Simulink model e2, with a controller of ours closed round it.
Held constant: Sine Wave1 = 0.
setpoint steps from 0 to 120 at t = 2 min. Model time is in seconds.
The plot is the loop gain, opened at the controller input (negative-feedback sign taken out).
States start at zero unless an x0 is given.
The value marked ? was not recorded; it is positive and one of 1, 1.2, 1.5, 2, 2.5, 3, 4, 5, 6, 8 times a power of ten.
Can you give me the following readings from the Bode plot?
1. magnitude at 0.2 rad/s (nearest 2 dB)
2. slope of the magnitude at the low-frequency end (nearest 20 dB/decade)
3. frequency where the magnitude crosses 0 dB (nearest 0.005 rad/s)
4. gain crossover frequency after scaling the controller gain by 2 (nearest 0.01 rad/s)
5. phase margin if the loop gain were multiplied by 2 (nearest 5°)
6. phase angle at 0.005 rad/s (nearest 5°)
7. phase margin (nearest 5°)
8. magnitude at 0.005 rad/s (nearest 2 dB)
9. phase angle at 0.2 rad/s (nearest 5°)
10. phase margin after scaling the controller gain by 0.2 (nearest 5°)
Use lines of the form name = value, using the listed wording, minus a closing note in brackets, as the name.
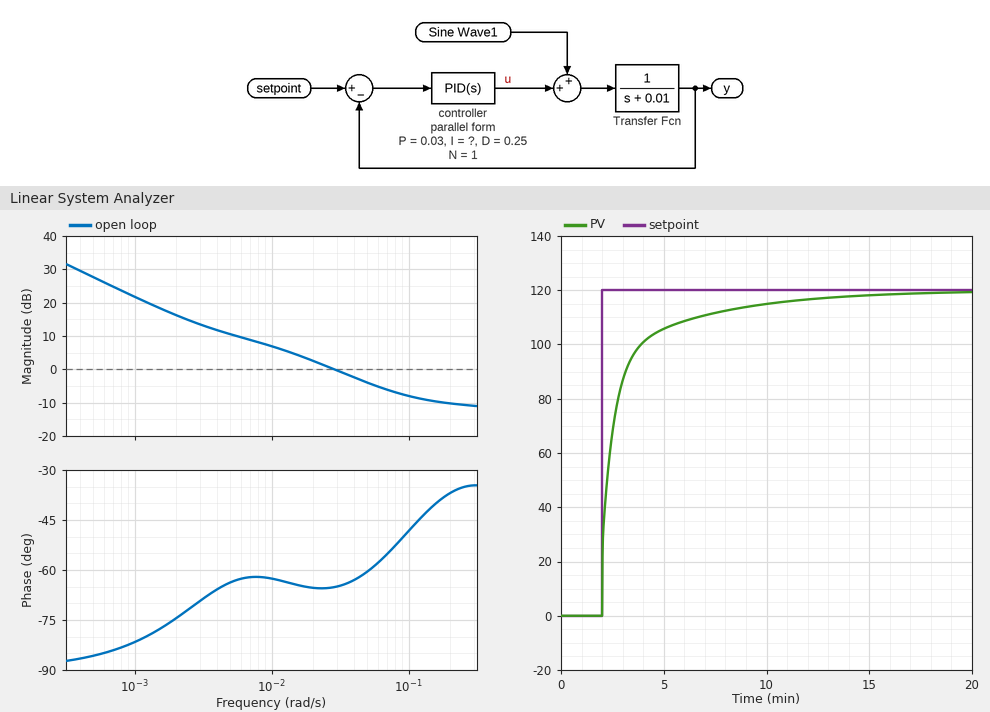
magnitude at 0.2 rad/s = -10 dB
slope of the magnitude at the low-frequency end = -20 dB/decade
frequency where the magnitude crosses 0 dB = 0.030 rad/s
gain crossover frequency after scaling the controller gain by 2 = 0.07 rad/s
phase margin if the loop gain were multiplied by 2 = 125°
phase angle at 0.005 rad/s = -65°
phase margin = 115°
magnitude at 0.005 rad/s = 10 dB
phase angle at 0.2 rad/s = -35°
phase margin after scaling the controller gain by 0.2 = 110°
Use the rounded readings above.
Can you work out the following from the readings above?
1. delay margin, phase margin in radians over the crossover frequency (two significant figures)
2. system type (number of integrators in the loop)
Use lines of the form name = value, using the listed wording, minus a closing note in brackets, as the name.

delay margin, phase margin in radians over the crossover frequency = 67 s
system type = 1
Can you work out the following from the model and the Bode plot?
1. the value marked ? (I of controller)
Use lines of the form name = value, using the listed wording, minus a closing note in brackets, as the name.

the value marked ? = 0.00012
